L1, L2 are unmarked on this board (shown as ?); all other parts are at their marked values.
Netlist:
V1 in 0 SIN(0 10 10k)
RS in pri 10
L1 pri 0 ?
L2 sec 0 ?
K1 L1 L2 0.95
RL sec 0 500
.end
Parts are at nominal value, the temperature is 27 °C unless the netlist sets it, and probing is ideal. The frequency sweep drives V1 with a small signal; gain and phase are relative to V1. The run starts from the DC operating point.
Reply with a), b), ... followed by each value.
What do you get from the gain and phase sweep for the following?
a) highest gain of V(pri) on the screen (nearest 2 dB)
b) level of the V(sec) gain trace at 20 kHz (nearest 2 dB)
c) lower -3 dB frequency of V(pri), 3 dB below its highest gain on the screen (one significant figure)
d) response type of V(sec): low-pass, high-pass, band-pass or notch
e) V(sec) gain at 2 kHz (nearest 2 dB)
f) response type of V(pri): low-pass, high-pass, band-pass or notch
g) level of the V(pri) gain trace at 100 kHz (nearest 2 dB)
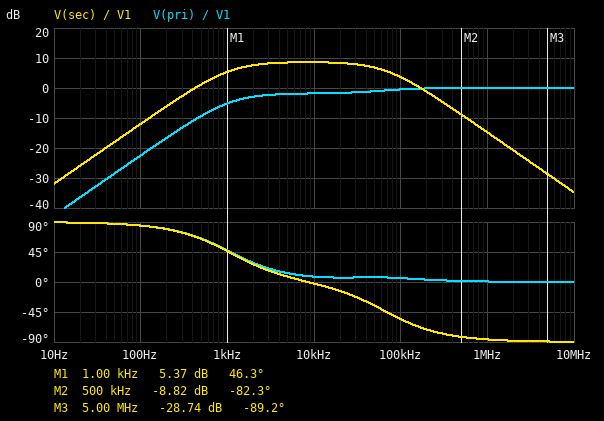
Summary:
a) 0 dB
b) 8 dB
c) 2 kHz
d) band-pass
e) 8 dB
f) high-pass
g) 0 dB
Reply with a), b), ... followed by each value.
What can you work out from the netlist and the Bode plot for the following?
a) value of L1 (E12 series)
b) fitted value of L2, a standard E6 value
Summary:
a) 1.2 mH
b) 15 mH
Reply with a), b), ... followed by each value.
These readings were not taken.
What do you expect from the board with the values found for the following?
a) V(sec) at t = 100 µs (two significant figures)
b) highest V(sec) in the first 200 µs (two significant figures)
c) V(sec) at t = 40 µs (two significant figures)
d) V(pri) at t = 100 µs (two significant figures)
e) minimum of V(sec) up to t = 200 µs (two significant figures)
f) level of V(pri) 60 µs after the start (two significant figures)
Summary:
a) -2.6 V
b) 26 V
c) 14 V
d) 700 mV
e) -29 V
f) -6.2 V
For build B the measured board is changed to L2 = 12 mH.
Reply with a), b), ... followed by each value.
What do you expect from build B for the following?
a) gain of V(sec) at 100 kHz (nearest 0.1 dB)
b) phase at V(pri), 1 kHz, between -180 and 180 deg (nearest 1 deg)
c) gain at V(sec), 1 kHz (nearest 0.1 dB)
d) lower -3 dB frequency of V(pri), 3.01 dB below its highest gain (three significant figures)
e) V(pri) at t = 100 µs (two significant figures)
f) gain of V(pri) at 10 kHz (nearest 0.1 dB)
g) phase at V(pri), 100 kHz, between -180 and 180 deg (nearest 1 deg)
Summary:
a) 4.0 dB
b) 48 deg
c) 4.6 dB
d) 1.71 kHz
e) 660 mV
f) -1.5 dB
g) 5 deg
